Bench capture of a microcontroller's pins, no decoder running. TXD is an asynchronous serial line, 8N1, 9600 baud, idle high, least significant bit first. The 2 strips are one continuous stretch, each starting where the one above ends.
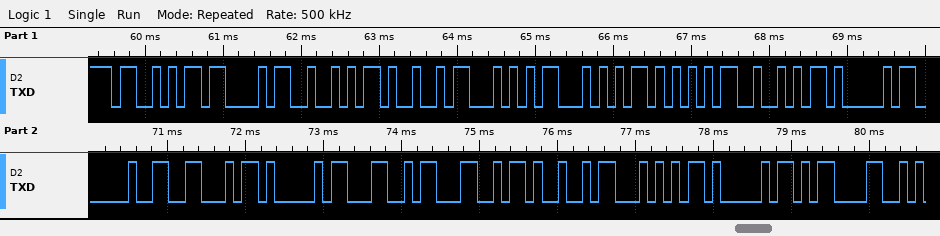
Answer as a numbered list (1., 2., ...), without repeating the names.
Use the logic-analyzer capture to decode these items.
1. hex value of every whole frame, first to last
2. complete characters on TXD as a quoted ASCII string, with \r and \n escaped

1. 53 43 52 49 54 54 55 52 41 20 46 41 4C 4C 49 54 41 0D
2. "SCRITTURA FALLITA\r"
